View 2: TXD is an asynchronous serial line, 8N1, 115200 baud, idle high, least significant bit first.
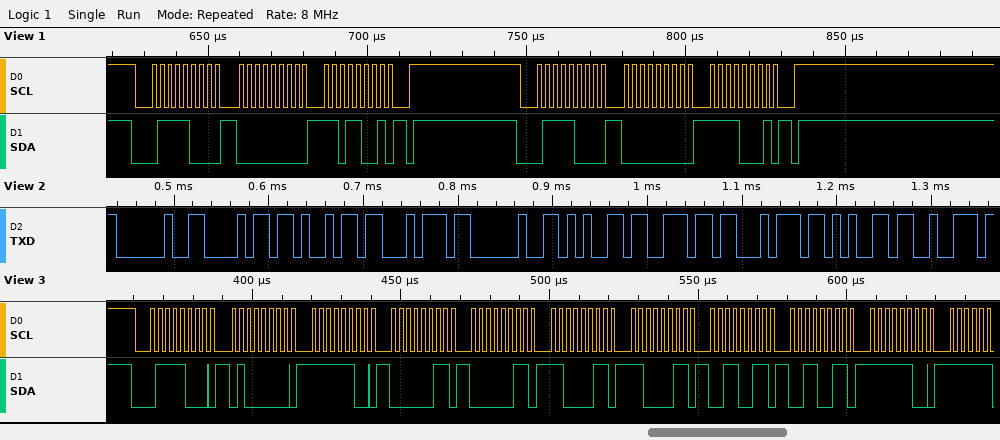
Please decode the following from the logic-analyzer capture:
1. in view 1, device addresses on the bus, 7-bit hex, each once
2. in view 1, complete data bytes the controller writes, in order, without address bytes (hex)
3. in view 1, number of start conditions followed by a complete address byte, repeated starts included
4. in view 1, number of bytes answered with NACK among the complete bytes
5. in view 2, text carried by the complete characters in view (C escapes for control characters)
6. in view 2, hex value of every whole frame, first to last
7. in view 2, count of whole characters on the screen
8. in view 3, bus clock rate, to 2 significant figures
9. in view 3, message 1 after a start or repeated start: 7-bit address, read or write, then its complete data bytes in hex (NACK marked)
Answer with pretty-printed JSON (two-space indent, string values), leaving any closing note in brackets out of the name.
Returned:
{
  "in view 1, device addresses on the bus, 7-bit hex, each once": "0x3C",
  "in view 1, complete data bytes the controller writes, in order, without address bytes": "00 D9 00 F1",
  "in view 1, number of start conditions followed by a complete address byte, repeated starts included": "2",
  "in view 1, number of bytes answered with NACK among the complete bytes": "0",
  "in view 2, text carried by the complete characters in view": "\" hit enter\"",
  "in view 2, hex value of every whole frame, first to last": "20 68 69 74 20 65 6E 74 65 72",
  "in view 2, count of whole characters on the screen": "10",
  "in view 3, bus clock rate, to 2 significant figures": "400 kHz",
  "in view 3, message 1 after a start or repeated start: 7-bit address, read or write, then its complete data bytes in hex": "0x3C write: 40 FC 03 03 C3 C3 33 33 FC"
}
